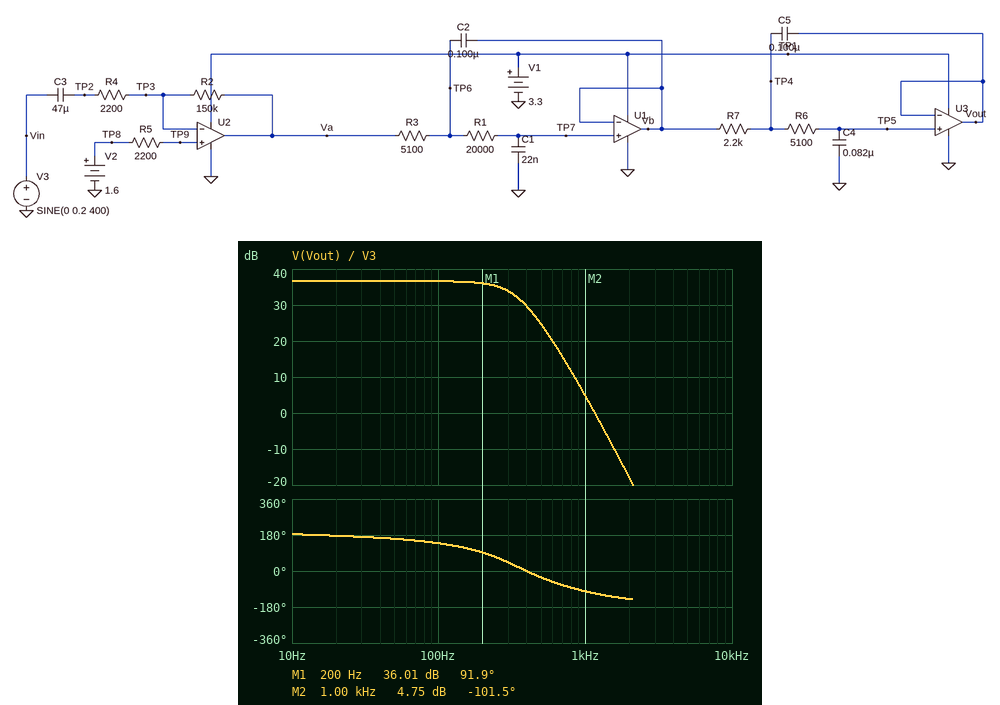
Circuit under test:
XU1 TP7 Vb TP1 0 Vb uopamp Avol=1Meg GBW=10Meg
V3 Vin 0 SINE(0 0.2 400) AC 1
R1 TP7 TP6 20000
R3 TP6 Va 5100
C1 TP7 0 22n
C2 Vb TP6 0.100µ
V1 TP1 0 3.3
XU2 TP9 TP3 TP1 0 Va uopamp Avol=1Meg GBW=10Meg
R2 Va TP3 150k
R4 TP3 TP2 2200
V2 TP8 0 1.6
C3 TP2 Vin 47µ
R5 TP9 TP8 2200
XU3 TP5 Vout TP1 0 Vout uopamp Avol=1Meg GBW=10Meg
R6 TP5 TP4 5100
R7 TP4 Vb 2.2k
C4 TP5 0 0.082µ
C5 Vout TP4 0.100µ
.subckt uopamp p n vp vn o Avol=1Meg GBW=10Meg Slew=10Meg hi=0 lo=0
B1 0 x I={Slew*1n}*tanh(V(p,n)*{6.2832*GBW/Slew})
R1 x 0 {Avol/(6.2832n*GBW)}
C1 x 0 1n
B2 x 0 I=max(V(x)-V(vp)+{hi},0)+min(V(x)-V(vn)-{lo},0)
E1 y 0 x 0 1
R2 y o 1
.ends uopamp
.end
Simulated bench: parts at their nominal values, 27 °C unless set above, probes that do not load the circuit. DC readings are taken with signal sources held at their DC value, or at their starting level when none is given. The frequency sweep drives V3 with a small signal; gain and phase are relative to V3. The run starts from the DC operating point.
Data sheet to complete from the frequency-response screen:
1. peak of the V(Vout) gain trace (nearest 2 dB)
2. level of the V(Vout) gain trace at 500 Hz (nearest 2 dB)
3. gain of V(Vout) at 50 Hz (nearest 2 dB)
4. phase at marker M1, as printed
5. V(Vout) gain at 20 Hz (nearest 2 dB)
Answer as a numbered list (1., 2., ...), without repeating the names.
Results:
1. 36 dB
2. 24 dB
3. 36 dB
4. 91.9 deg
5. 36 dB
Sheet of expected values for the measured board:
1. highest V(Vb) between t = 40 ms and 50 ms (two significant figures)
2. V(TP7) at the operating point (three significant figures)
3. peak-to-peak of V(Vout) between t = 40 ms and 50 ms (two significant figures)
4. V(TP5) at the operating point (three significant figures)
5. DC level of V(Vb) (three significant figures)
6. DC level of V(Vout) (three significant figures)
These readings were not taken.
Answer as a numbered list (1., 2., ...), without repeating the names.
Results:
1. 3.2 V
2. 1.60 V
3. 1.9 V
4. 1.60 V
5. 1.60 V
6. 1.60 V
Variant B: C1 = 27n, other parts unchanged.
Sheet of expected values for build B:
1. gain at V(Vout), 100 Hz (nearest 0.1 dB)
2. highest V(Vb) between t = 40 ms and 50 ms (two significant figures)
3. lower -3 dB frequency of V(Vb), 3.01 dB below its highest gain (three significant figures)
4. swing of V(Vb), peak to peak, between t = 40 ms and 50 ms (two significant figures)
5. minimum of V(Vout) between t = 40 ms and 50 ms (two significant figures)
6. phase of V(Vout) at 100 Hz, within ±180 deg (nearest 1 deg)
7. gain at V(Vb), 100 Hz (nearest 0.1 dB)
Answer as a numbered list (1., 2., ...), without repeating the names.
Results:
1. 36.5 dB
2. 2.8 V
3. 1.58 Hz
4. 2.4 V
5. 920 mV
6. 134 deg
7. 36.8 dB
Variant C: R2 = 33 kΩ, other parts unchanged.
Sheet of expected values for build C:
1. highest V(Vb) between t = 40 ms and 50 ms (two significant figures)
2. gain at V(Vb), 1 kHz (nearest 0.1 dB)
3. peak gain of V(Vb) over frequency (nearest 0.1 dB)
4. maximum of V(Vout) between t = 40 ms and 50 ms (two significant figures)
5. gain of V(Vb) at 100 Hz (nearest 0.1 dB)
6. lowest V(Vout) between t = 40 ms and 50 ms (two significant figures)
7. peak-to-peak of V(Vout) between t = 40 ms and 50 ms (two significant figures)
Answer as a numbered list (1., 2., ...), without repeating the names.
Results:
1. 3.0 V
2. 4.8 dB
3. 24.0 dB
4. 2.5 V
5. 23.7 dB
6. 750 mV
7. 1.8 V
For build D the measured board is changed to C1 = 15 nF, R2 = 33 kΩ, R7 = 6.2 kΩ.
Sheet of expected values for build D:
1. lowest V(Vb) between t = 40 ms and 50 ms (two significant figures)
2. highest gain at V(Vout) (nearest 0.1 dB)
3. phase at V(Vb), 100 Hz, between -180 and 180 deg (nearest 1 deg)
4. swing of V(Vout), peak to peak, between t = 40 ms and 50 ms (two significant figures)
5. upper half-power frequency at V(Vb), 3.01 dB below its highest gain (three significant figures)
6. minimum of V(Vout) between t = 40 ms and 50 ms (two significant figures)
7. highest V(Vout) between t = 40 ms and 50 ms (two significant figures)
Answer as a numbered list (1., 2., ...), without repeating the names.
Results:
1. -8.9 mV
2. 23.5 dB
3. 167 deg
4. 1.5 V
5. 478 Hz
6. 880 mV
7. 2.4 V
